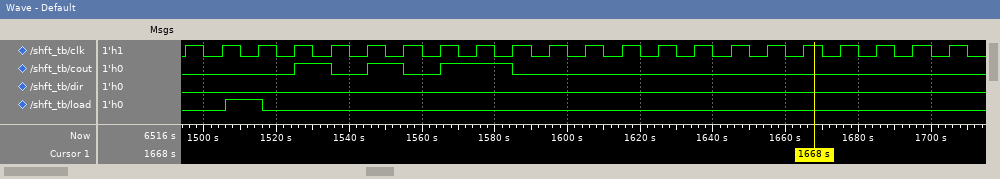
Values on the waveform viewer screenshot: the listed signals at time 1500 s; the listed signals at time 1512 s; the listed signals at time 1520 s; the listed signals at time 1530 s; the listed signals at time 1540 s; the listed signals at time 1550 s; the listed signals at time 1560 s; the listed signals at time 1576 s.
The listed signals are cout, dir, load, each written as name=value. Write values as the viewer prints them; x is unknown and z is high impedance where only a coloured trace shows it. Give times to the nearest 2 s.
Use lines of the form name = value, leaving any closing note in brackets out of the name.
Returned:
the listed signals at time 1500 s = cout=0, dir=0, load=0
the listed signals at time 1512 s = cout=0, dir=0, load=1
the listed signals at time 1520 s = cout=0, dir=0, load=0
the listed signals at time 1530 s = cout=1, dir=0, load=0
the listed signals at time 1540 s = cout=0, dir=0, load=0
the listed signals at time 1550 s = cout=1, dir=0, load=0
the listed signals at time 1560 s = cout=0, dir=0, load=0
the listed signals at time 1576 s = cout=1, dir=0, load=0
